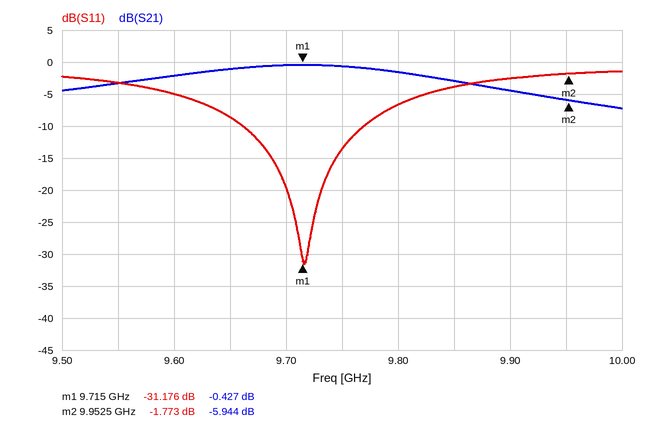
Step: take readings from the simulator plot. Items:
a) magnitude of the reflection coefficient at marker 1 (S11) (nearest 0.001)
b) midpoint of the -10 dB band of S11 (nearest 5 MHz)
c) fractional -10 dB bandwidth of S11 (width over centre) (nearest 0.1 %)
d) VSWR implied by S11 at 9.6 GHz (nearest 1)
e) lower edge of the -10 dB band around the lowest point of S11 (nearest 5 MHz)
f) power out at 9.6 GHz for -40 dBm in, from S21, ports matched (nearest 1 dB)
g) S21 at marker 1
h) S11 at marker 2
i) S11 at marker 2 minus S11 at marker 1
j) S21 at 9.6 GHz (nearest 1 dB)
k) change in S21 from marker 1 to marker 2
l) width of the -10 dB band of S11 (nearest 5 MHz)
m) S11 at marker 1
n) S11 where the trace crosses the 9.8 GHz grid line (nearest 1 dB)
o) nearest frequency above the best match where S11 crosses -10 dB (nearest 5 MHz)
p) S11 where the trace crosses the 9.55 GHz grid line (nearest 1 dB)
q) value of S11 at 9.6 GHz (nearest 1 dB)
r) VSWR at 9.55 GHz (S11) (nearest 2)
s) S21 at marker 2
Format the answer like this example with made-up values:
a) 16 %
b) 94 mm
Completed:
a) 0.028
b) 9.715 GHz
c) 1.1 %
d) 4
e) 9.660 GHz
f) -42 dBm
g) -0.427 dB
h) -1.773 dB
i) 29.403 dB
j) -2 dB
k) -5.517 dB
l) 110 MHz
m) -31.176 dB
n) -7 dB
o) 9.770 GHz
p) -3 dB
q) -5 dB
r) 6
s) -5.944 dB
